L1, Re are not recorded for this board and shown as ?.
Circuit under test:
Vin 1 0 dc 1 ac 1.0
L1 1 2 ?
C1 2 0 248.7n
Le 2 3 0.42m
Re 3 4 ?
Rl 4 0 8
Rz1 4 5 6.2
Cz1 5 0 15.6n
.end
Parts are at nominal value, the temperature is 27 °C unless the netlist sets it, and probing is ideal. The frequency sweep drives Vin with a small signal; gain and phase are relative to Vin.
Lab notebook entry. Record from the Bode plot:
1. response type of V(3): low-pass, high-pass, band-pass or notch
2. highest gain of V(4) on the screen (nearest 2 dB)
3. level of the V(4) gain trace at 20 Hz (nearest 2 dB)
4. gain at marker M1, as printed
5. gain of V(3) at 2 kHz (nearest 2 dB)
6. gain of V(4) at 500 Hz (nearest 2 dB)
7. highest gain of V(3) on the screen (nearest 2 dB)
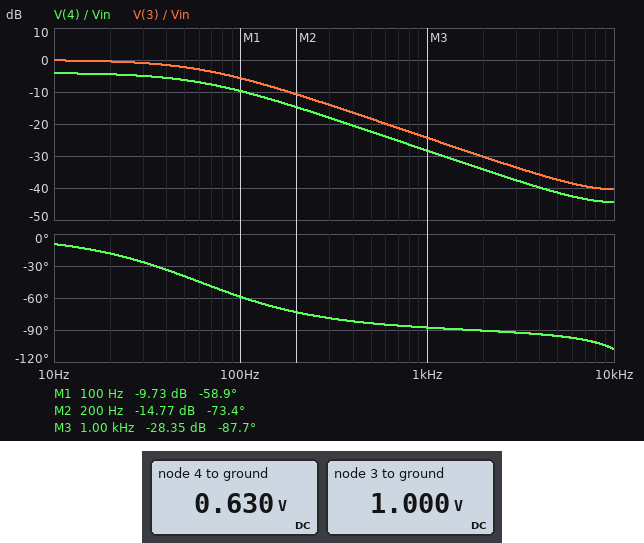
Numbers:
low-pass
-4 dB
-4 dB
-9.73 dB
-30 dB
-22 dB
0 dB
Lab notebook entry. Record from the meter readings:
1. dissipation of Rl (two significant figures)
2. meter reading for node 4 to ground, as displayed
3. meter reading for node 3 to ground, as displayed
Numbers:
50 mW
0.630 V
1.000 V
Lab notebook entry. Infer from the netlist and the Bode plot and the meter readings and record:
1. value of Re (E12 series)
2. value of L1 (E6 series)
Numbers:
4.7 Ω
33 mH
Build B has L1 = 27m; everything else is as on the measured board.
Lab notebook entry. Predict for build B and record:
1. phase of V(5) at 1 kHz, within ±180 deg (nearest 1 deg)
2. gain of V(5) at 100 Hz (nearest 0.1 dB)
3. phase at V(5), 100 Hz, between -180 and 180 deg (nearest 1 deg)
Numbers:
-87 deg
-8.5 dB
-54 deg
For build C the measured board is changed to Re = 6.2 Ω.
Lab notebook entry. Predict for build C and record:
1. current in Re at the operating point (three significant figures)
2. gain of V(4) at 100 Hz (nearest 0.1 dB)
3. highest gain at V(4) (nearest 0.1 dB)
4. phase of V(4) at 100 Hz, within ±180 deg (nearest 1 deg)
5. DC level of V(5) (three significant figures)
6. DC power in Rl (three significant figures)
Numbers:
70.4 mA
-10.0 dB
-5.0 dB
-56 deg
563 mV
39.7 mW
